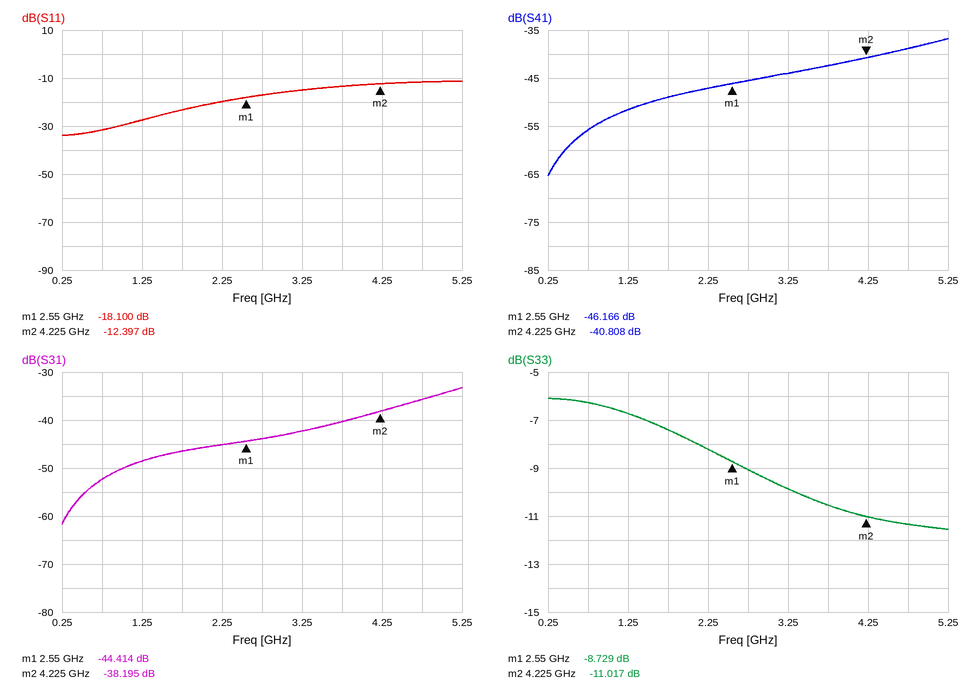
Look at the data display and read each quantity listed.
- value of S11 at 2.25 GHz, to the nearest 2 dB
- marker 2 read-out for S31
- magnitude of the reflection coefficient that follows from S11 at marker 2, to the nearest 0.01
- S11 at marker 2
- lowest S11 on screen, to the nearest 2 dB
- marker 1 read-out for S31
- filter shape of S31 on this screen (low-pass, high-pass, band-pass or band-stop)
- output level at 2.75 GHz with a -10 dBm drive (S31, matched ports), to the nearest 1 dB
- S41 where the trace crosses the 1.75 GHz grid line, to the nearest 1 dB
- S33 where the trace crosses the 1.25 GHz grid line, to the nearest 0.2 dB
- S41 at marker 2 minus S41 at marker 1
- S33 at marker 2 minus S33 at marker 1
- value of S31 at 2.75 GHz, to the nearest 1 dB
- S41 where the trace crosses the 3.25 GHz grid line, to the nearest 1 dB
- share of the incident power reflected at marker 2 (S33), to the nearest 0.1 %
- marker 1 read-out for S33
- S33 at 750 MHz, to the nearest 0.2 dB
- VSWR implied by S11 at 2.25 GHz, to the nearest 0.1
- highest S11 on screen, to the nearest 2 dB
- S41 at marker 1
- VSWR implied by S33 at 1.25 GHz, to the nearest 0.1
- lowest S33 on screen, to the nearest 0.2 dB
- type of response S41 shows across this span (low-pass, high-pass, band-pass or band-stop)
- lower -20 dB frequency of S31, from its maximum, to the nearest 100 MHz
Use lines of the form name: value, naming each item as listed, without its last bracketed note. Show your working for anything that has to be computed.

value of S11 at 2.25 GHz, to the nearest 2 dB: -20 dB
marker 2 read-out for S31: -38.195 dB
magnitude of the reflection coefficient that follows from S11 at marker 2, to the nearest 0.01: 10^(-12.397/20) ≈ 0.24
S11 at marker 2: -12.397 dB
lowest S11 on screen, to the nearest 2 dB: -34 dB
marker 1 read-out for S31: -44.414 dB
filter shape of S31 on this screen: high-pass
output level at 2.75 GHz with a -10 dBm drive (S31, matched ports), to the nearest 1 dB: -10 dBm + (-44 dB) = -54 dBm
S41 where the trace crosses the 1.75 GHz grid line, to the nearest 1 dB: -49 dB
S33 where the trace crosses the 1.25 GHz grid line, to the nearest 0.2 dB: -6.8 dB
S41 at marker 2 minus S41 at marker 1: -40.808 − (-46.166) = 5.358 dB
S33 at marker 2 minus S33 at marker 1: -11.017 − (-8.729) = -2.288 dB
value of S31 at 2.75 GHz, to the nearest 1 dB: -44 dB
S41 where the trace crosses the 3.25 GHz grid line, to the nearest 1 dB: -44 dB
share of the incident power reflected at marker 2 (S33), to the nearest 0.1 %: 10^(-11.017/10) ≈ 7.9 %
marker 1 read-out for S33: -8.729 dB
S33 at 750 MHz, to the nearest 0.2 dB: -6.2 dB
VSWR implied by S11 at 2.25 GHz, to the nearest 0.1: |Γ| = 10^(-20/20) = 0.1000; VSWR = (1 + 0.1000)/(1 − 0.1000) ≈ 1.2
highest S11 on screen, to the nearest 2 dB: -12 dB
S41 at marker 1: -46.166 dB
VSWR implied by S33 at 1.25 GHz, to the nearest 0.1: |Γ| = 10^(-6.8/20) = 0.4571; VSWR = (1 + 0.4571)/(1 − 0.4571) ≈ 2.7
lowest S33 on screen, to the nearest 0.2 dB: -11.6 dB
type of response S41 shows across this span: high-pass
lower -20 dB frequency of S31, from its maximum, to the nearest 100 MHz: 700 MHz
